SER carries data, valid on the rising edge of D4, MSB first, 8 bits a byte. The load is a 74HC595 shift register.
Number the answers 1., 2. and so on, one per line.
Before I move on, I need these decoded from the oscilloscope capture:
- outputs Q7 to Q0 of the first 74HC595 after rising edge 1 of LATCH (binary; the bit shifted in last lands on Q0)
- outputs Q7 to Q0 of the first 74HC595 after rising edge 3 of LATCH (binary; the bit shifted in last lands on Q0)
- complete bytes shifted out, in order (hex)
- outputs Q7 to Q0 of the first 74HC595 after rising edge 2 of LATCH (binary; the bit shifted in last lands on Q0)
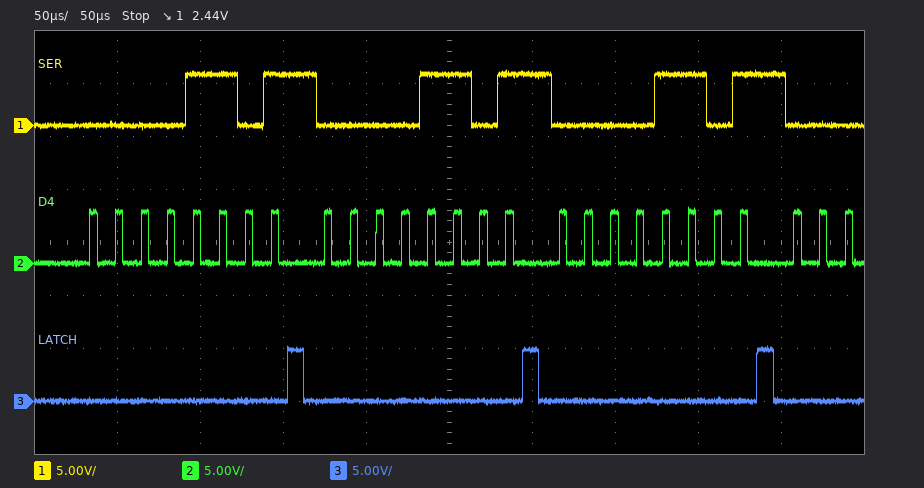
1. 00001101
2. 00001101
3. 0D 0D 0D
4. 00001101
